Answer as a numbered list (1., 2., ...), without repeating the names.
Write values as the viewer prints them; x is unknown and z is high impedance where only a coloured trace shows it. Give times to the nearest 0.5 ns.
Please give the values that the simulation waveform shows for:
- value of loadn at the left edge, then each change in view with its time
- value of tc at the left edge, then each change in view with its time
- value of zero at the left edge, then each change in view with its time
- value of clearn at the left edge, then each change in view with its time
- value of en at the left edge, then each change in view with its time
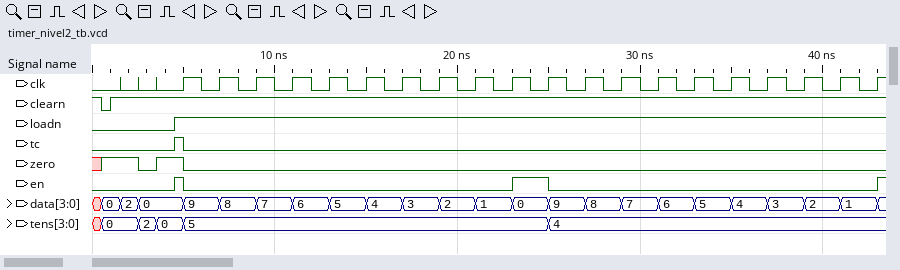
1. 0, 1 at 4.5 ns
2. 0, 1 at 4.5 ns, 0 at 5 ns
3. x, 1 at 0.5 ns, 0 at 2.5 ns, 1 at 3.5 ns, 0 at 5 ns
4. 1, 0 at 0.5 ns, 1 at 1 ns
5. 0, 1 at 4.5 ns, 0 at 5 ns, 1 at 23 ns, 0 at 25 ns, 1 at 43 ns
